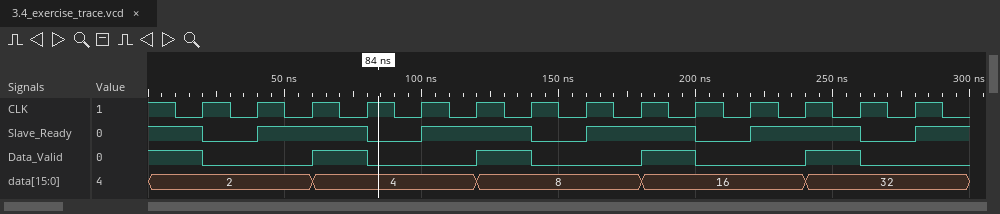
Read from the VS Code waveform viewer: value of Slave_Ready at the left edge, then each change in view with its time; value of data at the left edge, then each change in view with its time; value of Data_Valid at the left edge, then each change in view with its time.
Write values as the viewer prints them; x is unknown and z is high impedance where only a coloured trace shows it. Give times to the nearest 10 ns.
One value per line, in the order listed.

1, 0 at 20 ns, 1 at 40 ns, 0 at 80 ns, 1 at 100 ns, 0 at 140 ns, 1 at 160 ns, 0 at 200 ns, 1 at 220 ns, 0 at 260 ns, 1 at 280 ns
2, 4 at 60 ns, 8 at 120 ns, 16 at 180 ns, 32 at 240 ns
1, 0 at 20 ns, 1 at 60 ns, 0 at 80 ns, 1 at 120 ns, 0 at 140 ns, 1 at 180 ns, 0 at 200 ns, 1 at 240 ns, 0 at 260 ns
